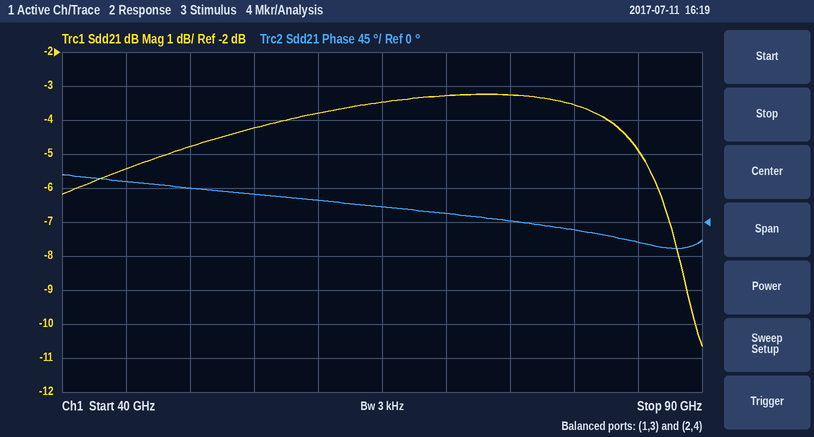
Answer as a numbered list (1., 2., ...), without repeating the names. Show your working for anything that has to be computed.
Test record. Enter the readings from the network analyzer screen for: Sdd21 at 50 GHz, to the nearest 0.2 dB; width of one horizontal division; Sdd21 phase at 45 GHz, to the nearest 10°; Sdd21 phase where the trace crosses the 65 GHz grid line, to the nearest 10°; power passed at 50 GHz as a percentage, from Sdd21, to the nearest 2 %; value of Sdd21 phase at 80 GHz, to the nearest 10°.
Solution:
1. -4.8 dB
2. 5 GHz
3. 50°
4. 20°
5. 10^(-4.8/10) ≈ 33.1 %, so 34 % to the nearest 2 %
6. -10°
